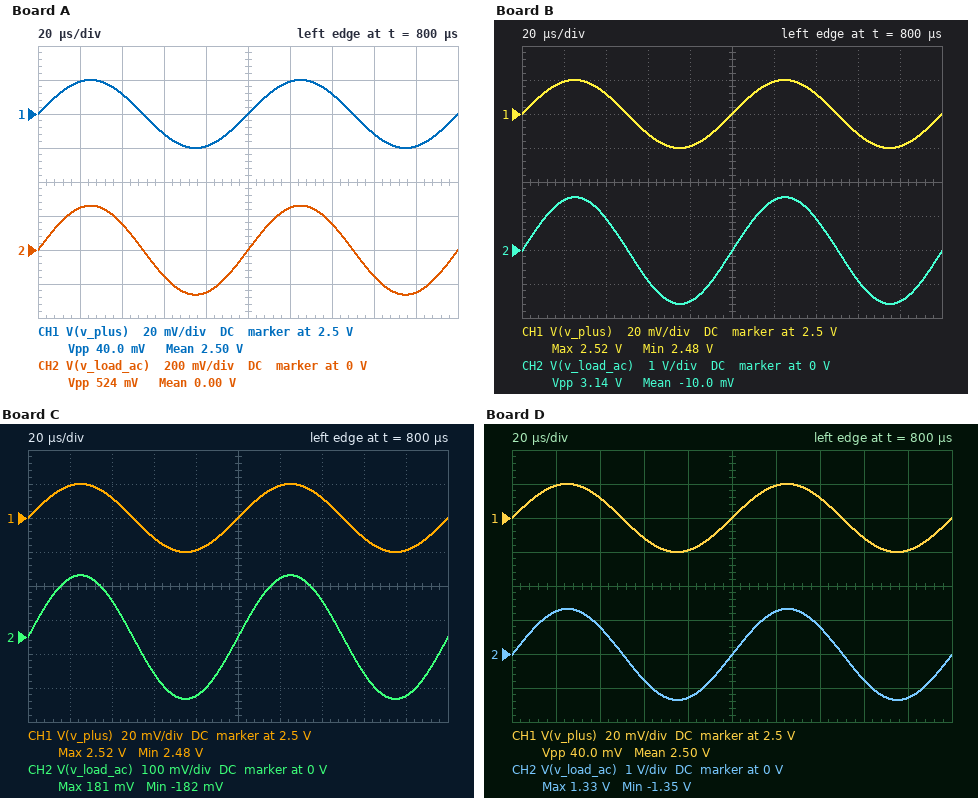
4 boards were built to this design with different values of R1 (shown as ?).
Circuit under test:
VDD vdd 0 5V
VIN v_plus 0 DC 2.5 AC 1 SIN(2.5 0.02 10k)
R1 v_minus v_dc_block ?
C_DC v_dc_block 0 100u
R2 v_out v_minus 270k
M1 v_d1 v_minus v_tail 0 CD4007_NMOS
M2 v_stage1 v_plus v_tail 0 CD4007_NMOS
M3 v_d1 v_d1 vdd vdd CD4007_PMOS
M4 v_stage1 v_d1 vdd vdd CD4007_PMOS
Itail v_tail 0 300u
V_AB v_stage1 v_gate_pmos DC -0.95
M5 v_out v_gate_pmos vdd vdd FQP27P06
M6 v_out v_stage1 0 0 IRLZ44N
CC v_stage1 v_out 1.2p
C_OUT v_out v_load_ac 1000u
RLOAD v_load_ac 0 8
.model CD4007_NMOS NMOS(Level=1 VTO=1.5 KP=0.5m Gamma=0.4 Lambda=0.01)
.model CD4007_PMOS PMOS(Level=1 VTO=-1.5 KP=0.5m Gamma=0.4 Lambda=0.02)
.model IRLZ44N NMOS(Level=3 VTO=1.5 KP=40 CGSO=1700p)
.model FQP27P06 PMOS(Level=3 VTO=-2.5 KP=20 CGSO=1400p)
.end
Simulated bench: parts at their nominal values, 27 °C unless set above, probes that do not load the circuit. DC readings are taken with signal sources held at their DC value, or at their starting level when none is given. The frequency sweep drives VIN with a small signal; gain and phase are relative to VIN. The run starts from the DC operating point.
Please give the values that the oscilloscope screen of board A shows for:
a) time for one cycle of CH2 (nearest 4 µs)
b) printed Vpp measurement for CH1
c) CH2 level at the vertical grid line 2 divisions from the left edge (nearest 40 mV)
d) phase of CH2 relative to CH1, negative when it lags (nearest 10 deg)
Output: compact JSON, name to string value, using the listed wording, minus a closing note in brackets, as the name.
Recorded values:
{"time for one cycle of CH2": "100 µs", "printed Vpp measurement for CH1": "40.0 mV", "CH2 level at the vertical grid line 2 divisions from the left edge": "160 mV", "phase of CH2 relative to CH1, negative when it lags": "0 deg"}
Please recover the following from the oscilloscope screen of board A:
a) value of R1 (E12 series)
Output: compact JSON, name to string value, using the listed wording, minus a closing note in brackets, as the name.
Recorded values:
{"value of R1": "22 kΩ"}
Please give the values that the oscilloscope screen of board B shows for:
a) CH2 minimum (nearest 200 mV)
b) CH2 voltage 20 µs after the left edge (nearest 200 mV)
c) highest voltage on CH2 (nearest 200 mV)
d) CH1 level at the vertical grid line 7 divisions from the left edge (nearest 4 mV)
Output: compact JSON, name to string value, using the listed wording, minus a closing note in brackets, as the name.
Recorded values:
{"CH2 minimum": "-1.6 V", "CH2 voltage 20 µs after the left edge": "1.4 V", "highest voltage on CH2": "1.6 V", "CH1 level at the vertical grid line 7 divisions from the left edge": "2.512 V"}
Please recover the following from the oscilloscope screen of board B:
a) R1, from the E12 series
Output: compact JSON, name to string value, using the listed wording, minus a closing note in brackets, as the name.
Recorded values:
{"R1, from the E12 series": "3.3 kΩ"}
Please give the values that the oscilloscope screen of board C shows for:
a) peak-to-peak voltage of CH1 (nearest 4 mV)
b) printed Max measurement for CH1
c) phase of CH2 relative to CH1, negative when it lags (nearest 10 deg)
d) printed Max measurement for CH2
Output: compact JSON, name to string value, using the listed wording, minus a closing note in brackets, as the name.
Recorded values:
{"peak-to-peak voltage of CH1": "40 mV", "printed Max measurement for CH1": "2.52 V", "phase of CH2 relative to CH1, negative when it lags": "0 deg", "printed Max measurement for CH2": "181 mV"}
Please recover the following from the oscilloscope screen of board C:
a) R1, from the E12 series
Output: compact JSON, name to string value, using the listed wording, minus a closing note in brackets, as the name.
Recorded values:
{"R1, from the E12 series": "33 kΩ"}
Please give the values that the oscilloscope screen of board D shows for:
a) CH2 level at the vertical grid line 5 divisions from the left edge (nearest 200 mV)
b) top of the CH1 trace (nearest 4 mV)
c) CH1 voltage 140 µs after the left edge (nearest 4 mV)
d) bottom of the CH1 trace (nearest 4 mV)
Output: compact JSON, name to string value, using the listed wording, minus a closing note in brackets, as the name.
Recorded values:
{"CH2 level at the vertical grid line 5 divisions from the left edge": "0 V", "top of the CH1 trace": "2.520 V", "CH1 voltage 140 µs after the left edge": "2.512 V", "bottom of the CH1 trace": "2.480 V"}
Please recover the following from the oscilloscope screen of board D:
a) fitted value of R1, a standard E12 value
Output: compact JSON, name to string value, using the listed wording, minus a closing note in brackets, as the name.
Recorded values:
{"fitted value of R1, a standard E12 value": "3.9 kΩ"}
